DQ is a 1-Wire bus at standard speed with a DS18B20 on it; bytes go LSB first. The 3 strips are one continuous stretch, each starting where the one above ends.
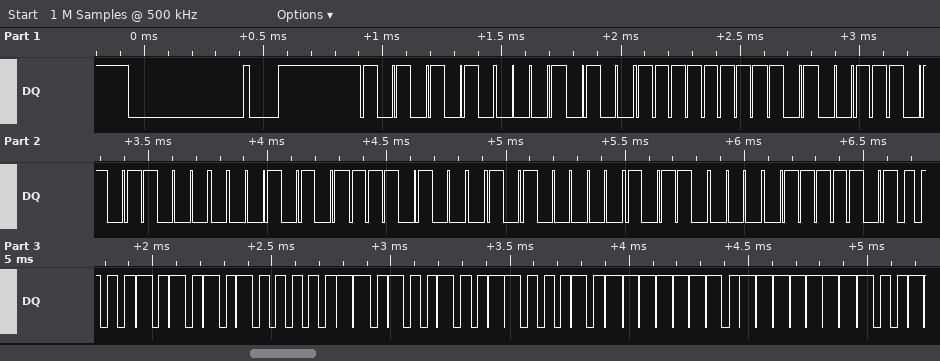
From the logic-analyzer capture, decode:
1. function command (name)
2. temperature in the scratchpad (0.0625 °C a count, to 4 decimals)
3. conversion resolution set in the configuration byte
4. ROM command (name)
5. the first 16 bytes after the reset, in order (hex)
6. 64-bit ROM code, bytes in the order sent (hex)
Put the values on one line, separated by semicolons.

Read Scratchpad; 85.0000 °C; 12 bits; Match ROM; 55 28 FF E5 1A A8 17 05 0D BE 50 05 4B 46 7F FF; 28 FF E5 1A A8 17 05 0D
